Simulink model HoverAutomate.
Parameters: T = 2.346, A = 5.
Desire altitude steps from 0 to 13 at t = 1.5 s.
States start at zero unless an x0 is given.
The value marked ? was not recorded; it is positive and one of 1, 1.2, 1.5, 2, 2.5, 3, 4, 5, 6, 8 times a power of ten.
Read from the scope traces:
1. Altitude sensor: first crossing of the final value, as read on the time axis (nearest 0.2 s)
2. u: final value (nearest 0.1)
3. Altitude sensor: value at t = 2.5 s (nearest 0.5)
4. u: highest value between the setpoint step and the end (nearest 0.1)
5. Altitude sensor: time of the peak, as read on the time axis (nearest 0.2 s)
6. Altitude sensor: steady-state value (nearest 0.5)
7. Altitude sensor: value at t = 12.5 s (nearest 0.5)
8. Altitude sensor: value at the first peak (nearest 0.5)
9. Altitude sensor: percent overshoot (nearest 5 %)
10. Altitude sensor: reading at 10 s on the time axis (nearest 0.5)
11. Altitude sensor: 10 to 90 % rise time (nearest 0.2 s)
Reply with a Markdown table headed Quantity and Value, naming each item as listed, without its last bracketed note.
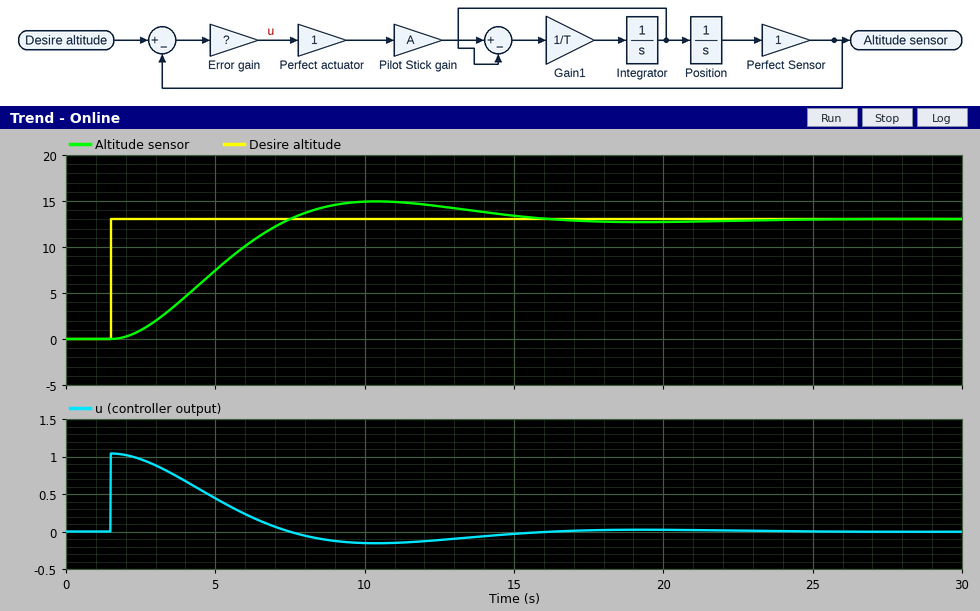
| Quantity | Value |
|---|---|
| Altitude sensor: first crossing of the final value, as read on the time axis | 7.4 s |
| u: final value | 0.0 |
| Altitude sensor: value at t = 2.5 s | 1.0 |
| u: highest value between the setpoint step and the end | 1.0 |
| Altitude sensor: time of the peak, as read on the time axis | 10.4 s |
| Altitude sensor: steady-state value | 13.0 |
| Altitude sensor: value at t = 12.5 s | 14.5 |
| Altitude sensor: value at the first peak | 15.0 |
| Altitude sensor: percent overshoot | 15 % |
| Altitude sensor: reading at 10 s on the time axis | 15.0 |
| Altitude sensor: 10 to 90 % rise time | 4.0 s |
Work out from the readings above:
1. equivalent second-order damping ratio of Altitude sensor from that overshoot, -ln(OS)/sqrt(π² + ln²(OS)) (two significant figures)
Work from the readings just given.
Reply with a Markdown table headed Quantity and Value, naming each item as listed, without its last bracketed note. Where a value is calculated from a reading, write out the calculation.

| Quantity | Value |
|---|---|
| equivalent second-order damping ratio of Altitude sensor from that overshoot, -ln(OS)/sqrt(π² + ln²(OS)) | ln(0.15) = -1.897; 1.897 / sqrt(9.870 + 3.599) = 0.52 |
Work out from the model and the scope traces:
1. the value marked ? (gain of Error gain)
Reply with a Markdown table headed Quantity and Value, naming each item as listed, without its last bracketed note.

| Quantity | Value |
|---|---|
| the value marked ? | 0.08 |
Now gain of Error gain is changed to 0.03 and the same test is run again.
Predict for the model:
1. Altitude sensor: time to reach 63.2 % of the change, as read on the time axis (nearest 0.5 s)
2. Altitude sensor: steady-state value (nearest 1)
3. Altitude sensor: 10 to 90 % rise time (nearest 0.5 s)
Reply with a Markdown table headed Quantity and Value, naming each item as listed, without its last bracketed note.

| Quantity | Value |
|---|---|
| Altitude sensor: time to reach 63.2 % of the change, as read on the time axis | 9.0 s |
| Altitude sensor: steady-state value | 13 |
| Altitude sensor: 10 to 90 % rise time | 10.5 s |
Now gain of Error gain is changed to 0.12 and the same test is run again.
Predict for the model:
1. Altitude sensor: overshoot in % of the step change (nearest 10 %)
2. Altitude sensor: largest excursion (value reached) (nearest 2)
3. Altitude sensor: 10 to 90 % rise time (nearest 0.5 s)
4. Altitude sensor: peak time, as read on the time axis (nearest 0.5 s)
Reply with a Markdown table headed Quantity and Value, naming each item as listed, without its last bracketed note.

| Quantity | Value |
|---|---|
| Altitude sensor: overshoot in % of the step change | 20 % |
| Altitude sensor: largest excursion (value reached) | 16 |
| Altitude sensor: 10 to 90 % rise time | 3.0 s |
| Altitude sensor: peak time, as read on the time axis | 8.5 s |
